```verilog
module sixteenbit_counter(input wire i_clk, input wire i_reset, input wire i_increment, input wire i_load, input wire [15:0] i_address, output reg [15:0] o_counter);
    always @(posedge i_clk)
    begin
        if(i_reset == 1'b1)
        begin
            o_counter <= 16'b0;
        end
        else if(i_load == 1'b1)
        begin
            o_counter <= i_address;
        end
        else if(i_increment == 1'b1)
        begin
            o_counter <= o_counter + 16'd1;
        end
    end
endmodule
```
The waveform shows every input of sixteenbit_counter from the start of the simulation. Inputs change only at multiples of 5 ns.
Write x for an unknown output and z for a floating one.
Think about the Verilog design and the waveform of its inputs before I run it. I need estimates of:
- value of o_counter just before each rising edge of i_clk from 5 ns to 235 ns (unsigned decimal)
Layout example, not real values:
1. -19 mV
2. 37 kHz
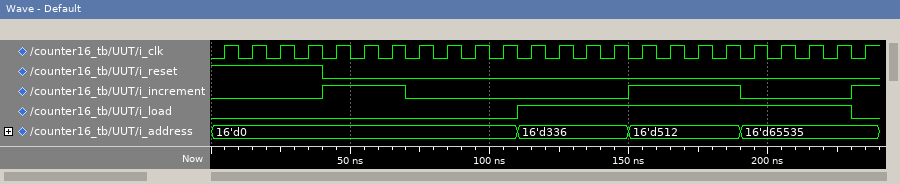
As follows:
1. x, 0, 0, 0, 0, 1, 2, 3, 3, 3, 3, 3, 336, 336, 336, 336, 512, 512, 512, 512, 65535, 65535, 65535, 65535
